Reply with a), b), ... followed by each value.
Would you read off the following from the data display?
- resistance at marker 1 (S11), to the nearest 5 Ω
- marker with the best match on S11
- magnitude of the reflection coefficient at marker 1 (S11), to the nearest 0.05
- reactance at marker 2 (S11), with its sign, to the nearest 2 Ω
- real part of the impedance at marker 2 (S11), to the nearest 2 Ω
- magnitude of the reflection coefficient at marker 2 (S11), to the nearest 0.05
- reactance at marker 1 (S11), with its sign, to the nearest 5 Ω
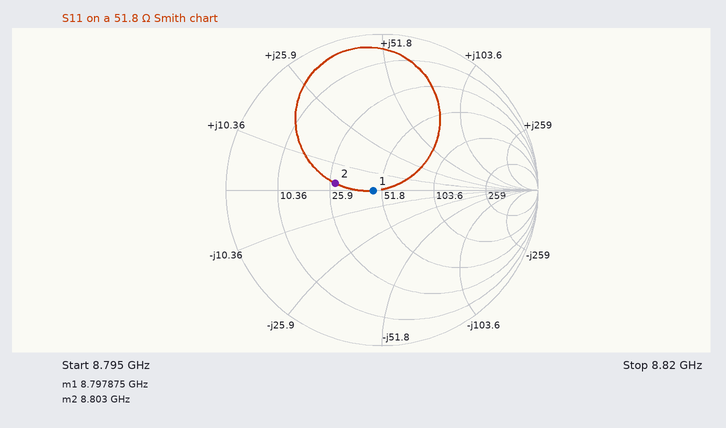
a) 45 Ω
b) marker 1
c) 0.05
d) +2 Ω
e) 28 Ω
f) 0.30
g) 0 Ω
